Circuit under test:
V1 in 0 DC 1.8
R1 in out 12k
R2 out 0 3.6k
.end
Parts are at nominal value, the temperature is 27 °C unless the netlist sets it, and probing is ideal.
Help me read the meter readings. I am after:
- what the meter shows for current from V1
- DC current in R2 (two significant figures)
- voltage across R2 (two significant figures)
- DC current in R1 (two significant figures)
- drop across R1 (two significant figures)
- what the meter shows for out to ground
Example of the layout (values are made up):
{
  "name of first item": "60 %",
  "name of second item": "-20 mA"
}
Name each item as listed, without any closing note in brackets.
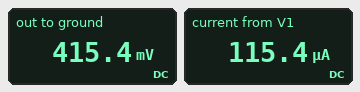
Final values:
{
  "what the meter shows for current from V1": "115.4 µA",
  "DC current in R2": "120 µA",
  "voltage across R2": "420 mV",
  "DC current in R1": "120 µA",
  "drop across R1": "1.4 V",
  "what the meter shows for out to ground": "415.4 mV"
}
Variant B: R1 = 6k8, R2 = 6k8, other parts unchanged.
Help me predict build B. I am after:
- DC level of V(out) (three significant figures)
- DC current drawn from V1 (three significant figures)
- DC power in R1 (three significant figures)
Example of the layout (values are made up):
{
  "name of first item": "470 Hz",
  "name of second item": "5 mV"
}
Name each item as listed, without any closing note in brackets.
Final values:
{
  "DC level of V(out)": "900 mV",
  "DC current drawn from V1": "132 µA",
  "DC power in R1": "119 µW"
}
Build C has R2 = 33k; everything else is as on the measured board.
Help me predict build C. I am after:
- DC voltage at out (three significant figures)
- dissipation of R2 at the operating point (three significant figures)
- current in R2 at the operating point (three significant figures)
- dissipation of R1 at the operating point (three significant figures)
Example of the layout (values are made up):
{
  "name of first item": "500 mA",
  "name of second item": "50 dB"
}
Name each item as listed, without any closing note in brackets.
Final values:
{
  "DC voltage at out": "1.32 V",
  "dissipation of R2 at the operating point": "52.8 µW",
  "current in R2 at the operating point": "40.0 µA",
  "dissipation of R1 at the operating point": "19.2 µW"
}
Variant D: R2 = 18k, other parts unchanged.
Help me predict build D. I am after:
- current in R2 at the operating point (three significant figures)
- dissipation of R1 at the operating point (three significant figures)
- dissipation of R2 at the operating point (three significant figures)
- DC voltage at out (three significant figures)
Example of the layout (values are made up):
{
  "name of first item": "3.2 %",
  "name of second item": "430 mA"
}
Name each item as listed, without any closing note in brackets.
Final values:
{
  "current in R2 at the operating point": "60.0 µA",
  "dissipation of R1 at the operating point": "43.2 µW",
  "dissipation of R2 at the operating point": "64.8 µW",
  "DC voltage at out": "1.08 V"
}
